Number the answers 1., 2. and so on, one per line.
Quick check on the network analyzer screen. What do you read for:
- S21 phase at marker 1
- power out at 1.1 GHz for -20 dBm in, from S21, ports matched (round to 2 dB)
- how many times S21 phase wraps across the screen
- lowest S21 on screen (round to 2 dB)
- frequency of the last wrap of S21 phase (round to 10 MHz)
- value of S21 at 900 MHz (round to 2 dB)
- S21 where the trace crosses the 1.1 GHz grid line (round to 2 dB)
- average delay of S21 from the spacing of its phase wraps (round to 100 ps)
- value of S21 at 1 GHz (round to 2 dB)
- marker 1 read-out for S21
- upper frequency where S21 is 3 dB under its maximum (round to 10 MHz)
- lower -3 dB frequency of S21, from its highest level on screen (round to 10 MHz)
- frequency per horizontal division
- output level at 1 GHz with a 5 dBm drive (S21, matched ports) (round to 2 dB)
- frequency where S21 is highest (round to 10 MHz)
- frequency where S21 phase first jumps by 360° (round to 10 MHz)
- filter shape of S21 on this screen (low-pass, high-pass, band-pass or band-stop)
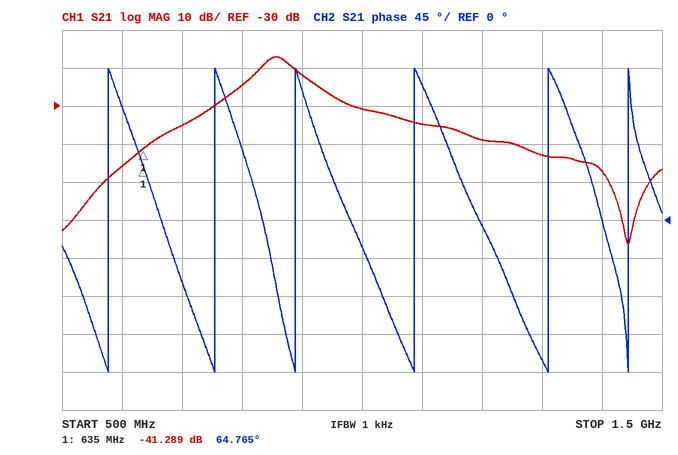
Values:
1. 64.765°
2. -54 dBm
3. 6
4. -66 dB
5. 1.44 GHz
6. -22 dB
7. -34 dB
8. 5.8 ns
9. -30 dB
10. -41.289 dB
11. 890 MHz
12. 830 MHz
13. 100 MHz
14. -26 dBm
15. 860 MHz
16. 580 MHz
17. band-pass
